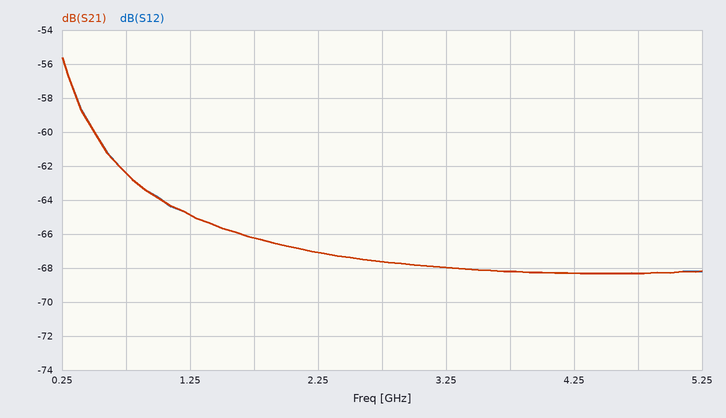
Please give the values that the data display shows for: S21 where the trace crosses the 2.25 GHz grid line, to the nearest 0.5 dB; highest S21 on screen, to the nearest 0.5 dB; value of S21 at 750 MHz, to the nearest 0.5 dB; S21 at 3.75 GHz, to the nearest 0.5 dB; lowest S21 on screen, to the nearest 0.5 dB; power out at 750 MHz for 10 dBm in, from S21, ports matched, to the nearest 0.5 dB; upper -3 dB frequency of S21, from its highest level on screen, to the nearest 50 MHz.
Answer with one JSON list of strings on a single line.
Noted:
["-67.0 dB", "-55.5 dB", "-62.5 dB", "-68.0 dB", "-68.5 dB", "-52.5 dBm", "400 MHz"]
